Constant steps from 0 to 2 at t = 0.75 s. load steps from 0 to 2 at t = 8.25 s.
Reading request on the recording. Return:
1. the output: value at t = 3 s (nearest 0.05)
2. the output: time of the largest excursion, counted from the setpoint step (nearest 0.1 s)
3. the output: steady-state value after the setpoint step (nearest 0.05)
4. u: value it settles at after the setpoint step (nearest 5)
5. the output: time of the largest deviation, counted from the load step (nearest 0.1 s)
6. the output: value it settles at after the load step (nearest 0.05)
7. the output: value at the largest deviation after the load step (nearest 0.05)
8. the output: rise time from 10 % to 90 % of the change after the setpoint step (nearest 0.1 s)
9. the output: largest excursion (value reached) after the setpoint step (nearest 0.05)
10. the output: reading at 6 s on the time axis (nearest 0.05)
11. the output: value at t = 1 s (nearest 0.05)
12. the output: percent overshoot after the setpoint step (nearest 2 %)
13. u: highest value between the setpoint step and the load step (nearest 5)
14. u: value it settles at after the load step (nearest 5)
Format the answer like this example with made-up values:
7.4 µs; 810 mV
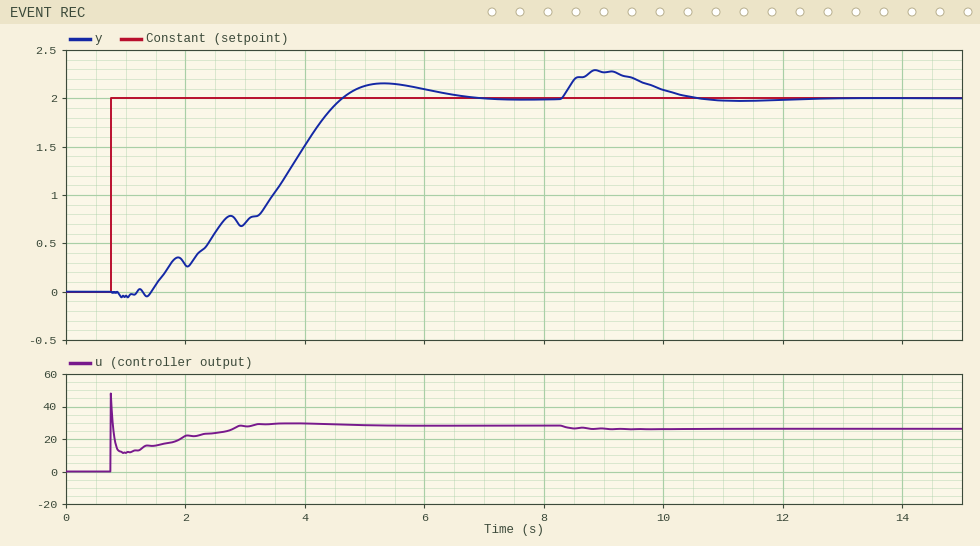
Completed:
0.70; 4.6 s; 2.00; 30; 0.6 s; 2.00; 2.30; 2.7 s; 2.15; 2.10; -0.05; 8 %; 50; 25
